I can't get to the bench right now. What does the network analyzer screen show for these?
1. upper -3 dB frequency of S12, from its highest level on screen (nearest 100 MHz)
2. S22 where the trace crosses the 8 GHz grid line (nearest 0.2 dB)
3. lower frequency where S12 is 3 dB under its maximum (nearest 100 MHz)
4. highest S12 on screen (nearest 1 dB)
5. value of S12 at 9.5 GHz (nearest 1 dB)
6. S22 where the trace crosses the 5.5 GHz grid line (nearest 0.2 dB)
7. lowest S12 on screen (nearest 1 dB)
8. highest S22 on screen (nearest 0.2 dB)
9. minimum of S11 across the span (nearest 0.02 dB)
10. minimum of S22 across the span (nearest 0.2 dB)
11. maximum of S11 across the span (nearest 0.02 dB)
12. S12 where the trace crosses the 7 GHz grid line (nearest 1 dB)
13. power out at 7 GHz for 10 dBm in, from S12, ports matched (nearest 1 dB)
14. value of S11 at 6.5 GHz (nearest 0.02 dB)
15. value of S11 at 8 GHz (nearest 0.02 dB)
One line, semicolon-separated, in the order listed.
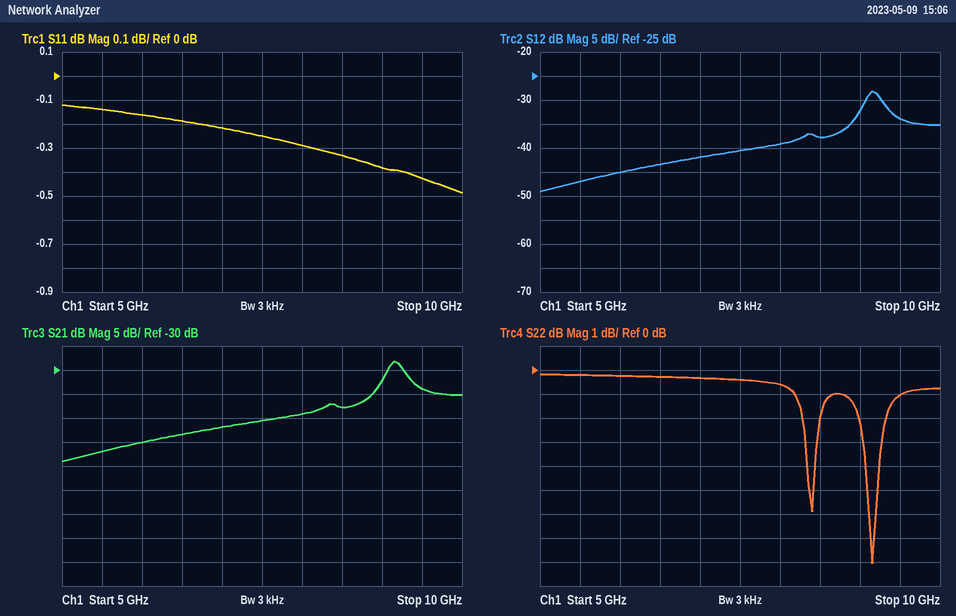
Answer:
9.3 GHz; -0.6 dB; 9.0 GHz; -28 dB; -34 dB; -0.2 dB; -49 dB; -0.2 dB; -0.48 dB; -8.0 dB; -0.12 dB; -42 dB; -32 dBm; -0.18 dB; -0.28 dB
